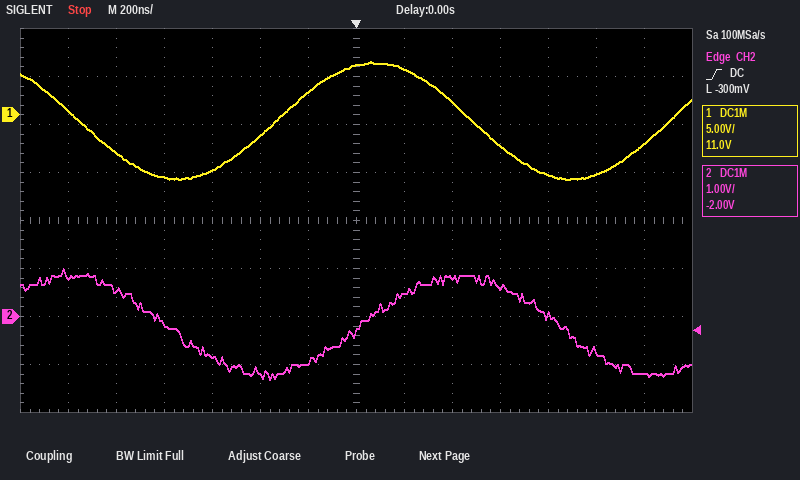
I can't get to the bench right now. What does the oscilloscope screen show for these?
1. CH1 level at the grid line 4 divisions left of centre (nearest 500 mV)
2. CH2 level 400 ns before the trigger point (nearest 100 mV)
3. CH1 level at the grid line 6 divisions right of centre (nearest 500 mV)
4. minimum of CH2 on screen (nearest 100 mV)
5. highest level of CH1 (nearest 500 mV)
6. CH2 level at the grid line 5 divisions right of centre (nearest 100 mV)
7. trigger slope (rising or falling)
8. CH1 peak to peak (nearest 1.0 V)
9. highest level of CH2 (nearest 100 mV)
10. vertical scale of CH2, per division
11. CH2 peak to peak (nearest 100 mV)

-6.5 V
-1.2 V
-3.0 V
-1.3 V
5.5 V
-700 mV
rising
12.0 V
1.0 V
1 V
2.3 V
